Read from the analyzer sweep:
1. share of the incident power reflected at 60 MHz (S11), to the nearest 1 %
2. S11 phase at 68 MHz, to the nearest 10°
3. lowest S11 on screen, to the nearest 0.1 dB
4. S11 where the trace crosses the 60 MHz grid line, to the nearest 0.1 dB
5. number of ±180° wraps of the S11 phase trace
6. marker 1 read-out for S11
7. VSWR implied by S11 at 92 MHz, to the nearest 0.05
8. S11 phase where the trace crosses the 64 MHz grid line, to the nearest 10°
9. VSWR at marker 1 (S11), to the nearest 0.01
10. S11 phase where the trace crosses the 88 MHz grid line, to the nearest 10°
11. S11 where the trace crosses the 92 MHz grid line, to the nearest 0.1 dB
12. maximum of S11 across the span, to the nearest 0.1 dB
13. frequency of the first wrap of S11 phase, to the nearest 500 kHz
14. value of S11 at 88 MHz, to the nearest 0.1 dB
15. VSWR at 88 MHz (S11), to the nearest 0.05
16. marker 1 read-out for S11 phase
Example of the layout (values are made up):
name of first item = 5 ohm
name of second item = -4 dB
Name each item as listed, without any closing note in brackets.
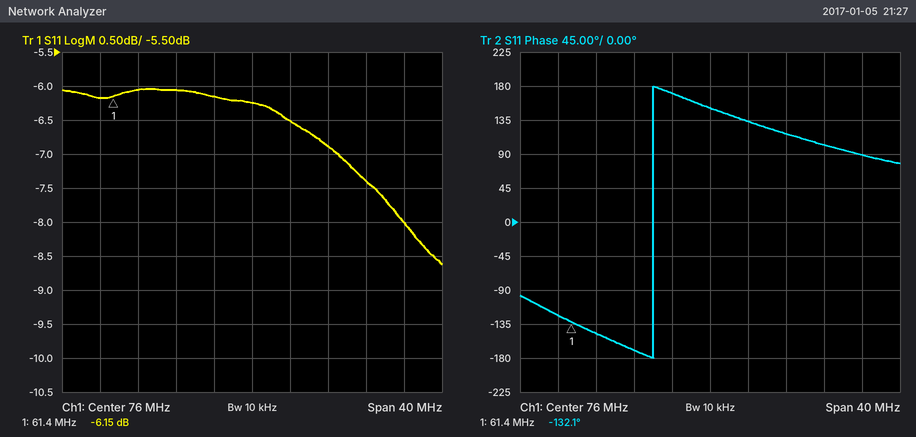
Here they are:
share of the incident power reflected at 60 MHz (S11), to the nearest 1 % = 24 %
S11 phase at 68 MHz, to the nearest 10° = -170°
lowest S11 on screen, to the nearest 0.1 dB = -8.6 dB
S11 where the trace crosses the 60 MHz grid line, to the nearest 0.1 dB = -6.2 dB
number of ±180° wraps of the S11 phase trace = 1
marker 1 read-out for S11 = -6.15 dB
VSWR implied by S11 at 92 MHz, to the nearest 0.05 = 2.30
S11 phase where the trace crosses the 64 MHz grid line, to the nearest 10° = -150°
VSWR at marker 1 (S11), to the nearest 0.01 = 2.94
S11 phase where the trace crosses the 88 MHz grid line, to the nearest 10° = 100°
S11 where the trace crosses the 92 MHz grid line, to the nearest 0.1 dB = -8.0 dB
maximum of S11 across the span, to the nearest 0.1 dB = -6.0 dB
frequency of the first wrap of S11 phase, to the nearest 500 kHz = 70.0 MHz
value of S11 at 88 MHz, to the nearest 0.1 dB = -7.4 dB
VSWR at 88 MHz (S11), to the nearest 0.05 = 2.50
marker 1 read-out for S11 phase = -132.1°
